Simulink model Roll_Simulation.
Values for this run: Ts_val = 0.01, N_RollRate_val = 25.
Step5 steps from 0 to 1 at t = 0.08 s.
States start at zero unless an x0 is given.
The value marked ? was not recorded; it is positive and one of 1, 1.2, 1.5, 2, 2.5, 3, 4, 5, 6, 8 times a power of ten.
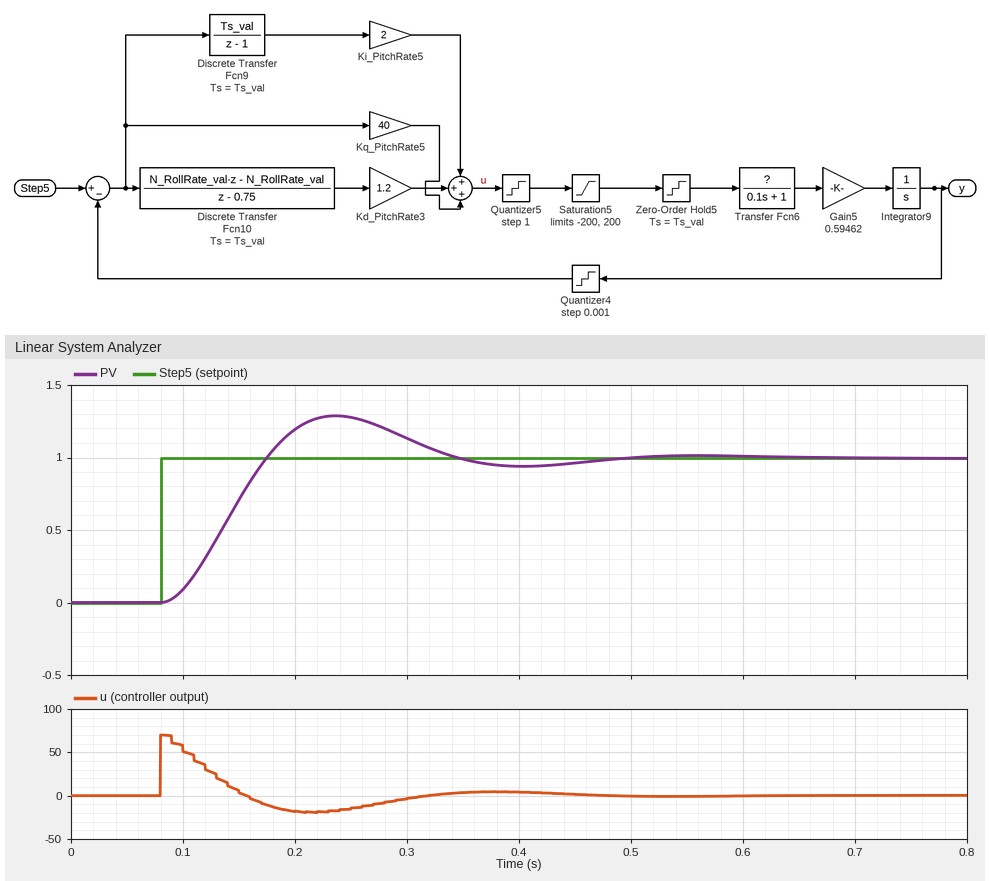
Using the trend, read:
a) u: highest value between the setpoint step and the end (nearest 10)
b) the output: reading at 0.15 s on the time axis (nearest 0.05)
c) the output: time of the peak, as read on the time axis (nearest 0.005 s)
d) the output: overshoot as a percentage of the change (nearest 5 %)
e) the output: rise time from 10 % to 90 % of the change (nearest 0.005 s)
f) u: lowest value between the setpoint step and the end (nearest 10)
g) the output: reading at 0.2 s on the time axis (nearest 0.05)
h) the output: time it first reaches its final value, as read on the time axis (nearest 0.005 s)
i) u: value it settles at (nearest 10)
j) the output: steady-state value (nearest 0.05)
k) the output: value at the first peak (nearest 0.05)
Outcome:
70
0.70
0.235 s
30 %
0.065 s
-20
1.20
0.175 s
0
1.00
1.30
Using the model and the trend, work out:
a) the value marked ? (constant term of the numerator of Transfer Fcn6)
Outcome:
1.2
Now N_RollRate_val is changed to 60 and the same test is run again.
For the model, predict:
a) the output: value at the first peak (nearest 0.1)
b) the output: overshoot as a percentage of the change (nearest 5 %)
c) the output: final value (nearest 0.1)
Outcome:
1.2
20 %
1.0
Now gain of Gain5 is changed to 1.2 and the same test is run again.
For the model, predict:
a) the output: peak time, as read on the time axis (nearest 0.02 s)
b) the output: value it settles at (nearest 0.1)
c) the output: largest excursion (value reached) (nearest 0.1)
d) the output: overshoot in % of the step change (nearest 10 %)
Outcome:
0.18 s
1.0
1.5
50 %
